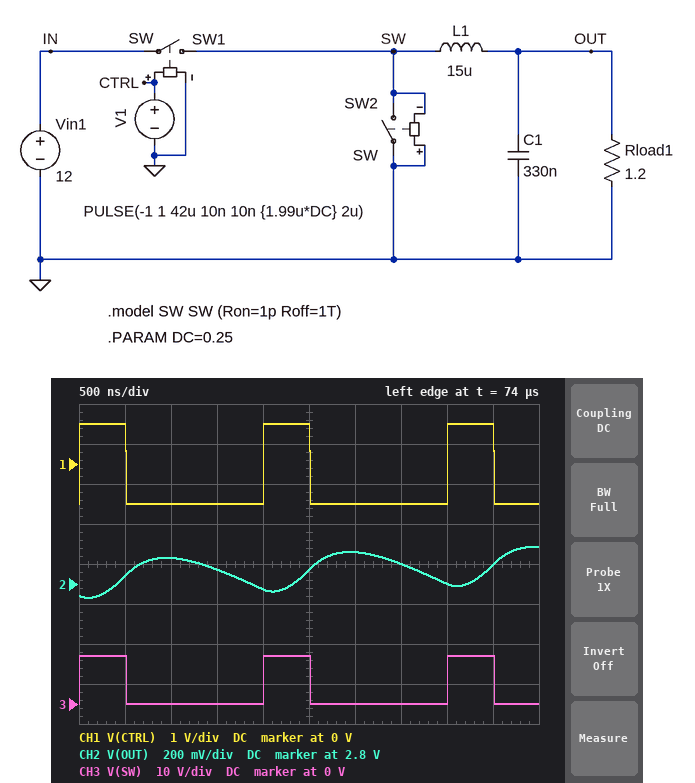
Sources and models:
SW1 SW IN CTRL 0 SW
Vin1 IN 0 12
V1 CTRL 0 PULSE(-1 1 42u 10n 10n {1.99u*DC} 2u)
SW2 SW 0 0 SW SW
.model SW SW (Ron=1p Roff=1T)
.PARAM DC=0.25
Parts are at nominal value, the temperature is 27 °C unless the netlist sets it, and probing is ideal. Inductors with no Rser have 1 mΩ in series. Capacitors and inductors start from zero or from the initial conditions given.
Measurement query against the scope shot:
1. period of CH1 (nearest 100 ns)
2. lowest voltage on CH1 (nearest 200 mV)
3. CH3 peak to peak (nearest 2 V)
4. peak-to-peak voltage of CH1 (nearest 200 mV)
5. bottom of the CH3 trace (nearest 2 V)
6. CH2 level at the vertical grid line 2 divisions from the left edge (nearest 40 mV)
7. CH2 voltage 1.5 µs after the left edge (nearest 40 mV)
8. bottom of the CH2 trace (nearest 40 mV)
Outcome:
2.0 µs
-1.0 V
12 V
2.0 V
0 V
2.92 V
2.88 V
2.72 V
